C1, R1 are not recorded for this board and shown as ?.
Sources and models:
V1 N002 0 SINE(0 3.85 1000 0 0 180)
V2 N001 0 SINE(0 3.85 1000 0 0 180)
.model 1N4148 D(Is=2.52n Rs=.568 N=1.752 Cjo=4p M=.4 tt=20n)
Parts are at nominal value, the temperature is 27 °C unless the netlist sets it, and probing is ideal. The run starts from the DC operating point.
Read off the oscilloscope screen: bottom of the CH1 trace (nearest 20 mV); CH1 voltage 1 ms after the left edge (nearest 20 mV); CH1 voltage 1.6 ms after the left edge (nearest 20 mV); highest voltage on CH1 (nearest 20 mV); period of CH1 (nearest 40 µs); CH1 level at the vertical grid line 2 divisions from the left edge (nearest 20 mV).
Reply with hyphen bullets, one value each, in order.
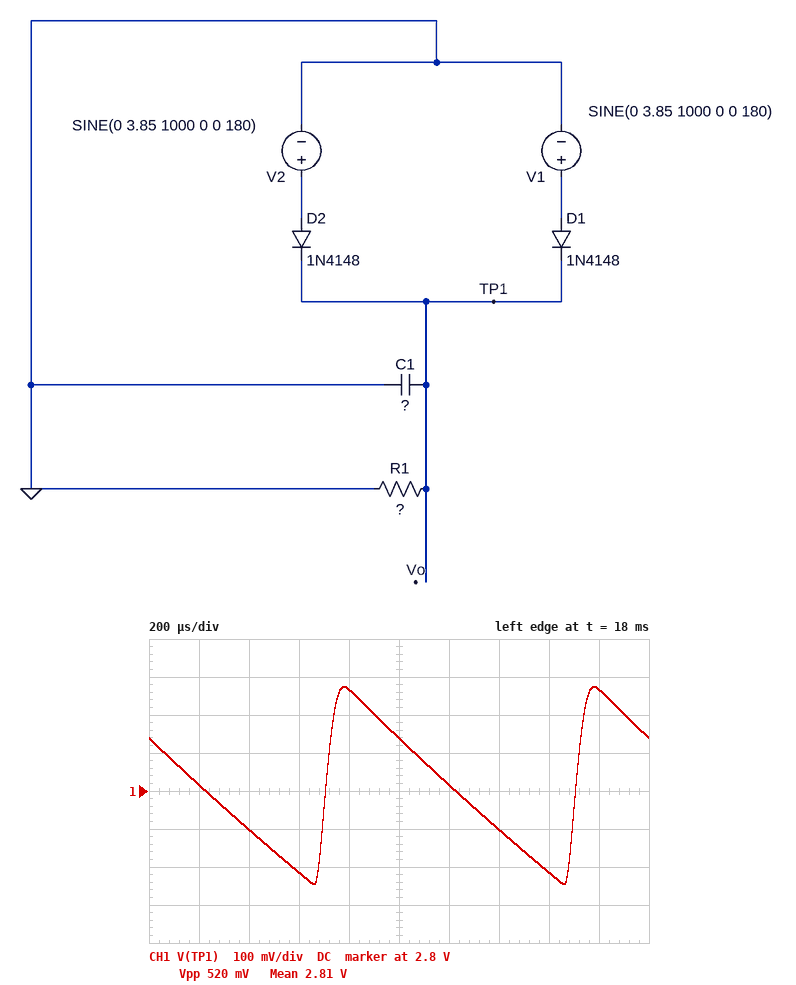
- 2.56 V
- 2.94 V
- 2.58 V
- 3.08 V
- 1.00 ms
- 2.70 V
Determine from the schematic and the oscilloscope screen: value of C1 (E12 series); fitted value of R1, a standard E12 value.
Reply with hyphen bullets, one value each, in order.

- 39 µF
- 120 Ω
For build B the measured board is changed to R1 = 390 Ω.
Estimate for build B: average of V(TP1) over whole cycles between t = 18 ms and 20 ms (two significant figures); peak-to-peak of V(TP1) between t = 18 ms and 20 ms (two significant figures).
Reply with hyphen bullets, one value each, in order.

- 3.0 V
- 180 mV
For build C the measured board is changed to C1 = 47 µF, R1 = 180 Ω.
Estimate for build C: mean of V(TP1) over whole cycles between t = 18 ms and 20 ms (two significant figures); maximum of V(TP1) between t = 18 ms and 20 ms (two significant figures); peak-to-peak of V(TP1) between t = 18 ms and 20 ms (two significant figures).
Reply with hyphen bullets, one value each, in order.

- 2.9 V
- 3.1 V
- 300 mV
